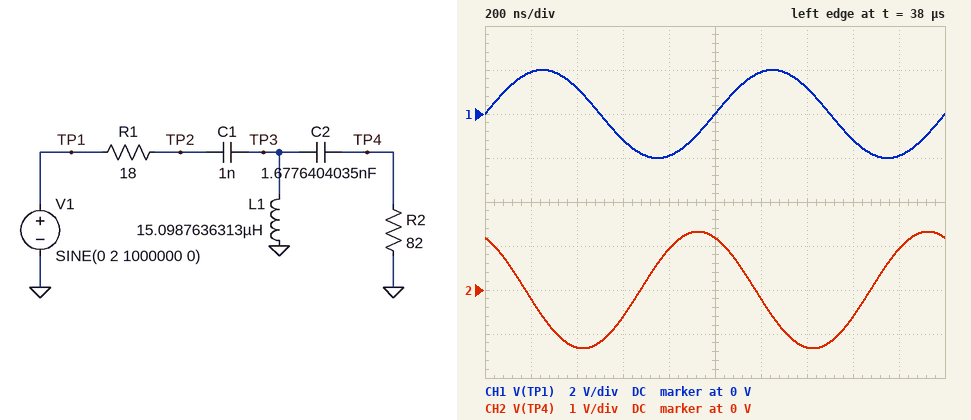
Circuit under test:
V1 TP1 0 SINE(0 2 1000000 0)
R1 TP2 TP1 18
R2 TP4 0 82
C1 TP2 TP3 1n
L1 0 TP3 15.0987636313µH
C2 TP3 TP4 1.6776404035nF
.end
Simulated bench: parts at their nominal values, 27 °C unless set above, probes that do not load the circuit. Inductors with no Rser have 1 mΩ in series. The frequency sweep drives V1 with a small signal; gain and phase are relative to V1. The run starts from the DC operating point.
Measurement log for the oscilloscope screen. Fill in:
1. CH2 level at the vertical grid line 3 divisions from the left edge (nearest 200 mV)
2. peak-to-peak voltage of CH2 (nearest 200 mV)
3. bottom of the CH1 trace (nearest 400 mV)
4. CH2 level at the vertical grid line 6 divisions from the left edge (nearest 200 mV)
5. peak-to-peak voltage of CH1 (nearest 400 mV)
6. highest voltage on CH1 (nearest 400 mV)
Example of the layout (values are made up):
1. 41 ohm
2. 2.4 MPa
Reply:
1. -600 mV
2. 2.6 V
3. -2.0 V
4. -200 mV
5. 4.0 V
6. 2.0 V
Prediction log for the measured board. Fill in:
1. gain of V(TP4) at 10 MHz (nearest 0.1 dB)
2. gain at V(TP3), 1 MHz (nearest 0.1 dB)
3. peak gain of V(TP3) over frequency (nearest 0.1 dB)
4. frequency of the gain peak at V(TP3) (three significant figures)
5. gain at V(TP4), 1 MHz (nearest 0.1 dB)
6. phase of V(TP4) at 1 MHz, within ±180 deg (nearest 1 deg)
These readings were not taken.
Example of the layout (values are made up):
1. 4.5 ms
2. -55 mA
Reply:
1. -1.9 dB
2. 0.1 dB
3. 0.7 dB
4. 888 kHz
5. -3.6 dB
6. 117 deg
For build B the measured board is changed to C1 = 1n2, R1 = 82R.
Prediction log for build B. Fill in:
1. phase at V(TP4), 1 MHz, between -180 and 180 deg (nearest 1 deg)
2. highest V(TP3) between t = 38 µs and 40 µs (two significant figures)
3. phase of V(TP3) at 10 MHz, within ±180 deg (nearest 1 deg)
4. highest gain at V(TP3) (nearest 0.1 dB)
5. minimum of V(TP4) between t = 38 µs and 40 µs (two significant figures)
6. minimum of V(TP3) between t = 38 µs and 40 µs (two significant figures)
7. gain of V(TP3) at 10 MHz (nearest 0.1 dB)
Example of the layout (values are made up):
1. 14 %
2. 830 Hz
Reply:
1. 101 deg
2. 1.5 V
3. 4 deg
4. -1.9 dB
5. -970 mV
6. -1.5 V
7. -6.0 dB
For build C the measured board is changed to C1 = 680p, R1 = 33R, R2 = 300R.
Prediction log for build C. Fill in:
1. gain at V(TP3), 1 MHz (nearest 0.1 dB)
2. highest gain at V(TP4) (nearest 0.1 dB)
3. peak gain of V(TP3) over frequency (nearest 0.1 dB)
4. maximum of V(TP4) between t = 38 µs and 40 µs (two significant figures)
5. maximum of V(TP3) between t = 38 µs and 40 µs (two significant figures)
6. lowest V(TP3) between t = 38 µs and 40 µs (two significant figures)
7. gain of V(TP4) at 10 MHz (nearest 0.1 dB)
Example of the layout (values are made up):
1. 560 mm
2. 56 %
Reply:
1. -3.7 dB
2. 2.9 dB
3. 3.0 dB
4. 1.2 V
5. 1.3 V
6. -1.3 V
7. -0.8 dB
